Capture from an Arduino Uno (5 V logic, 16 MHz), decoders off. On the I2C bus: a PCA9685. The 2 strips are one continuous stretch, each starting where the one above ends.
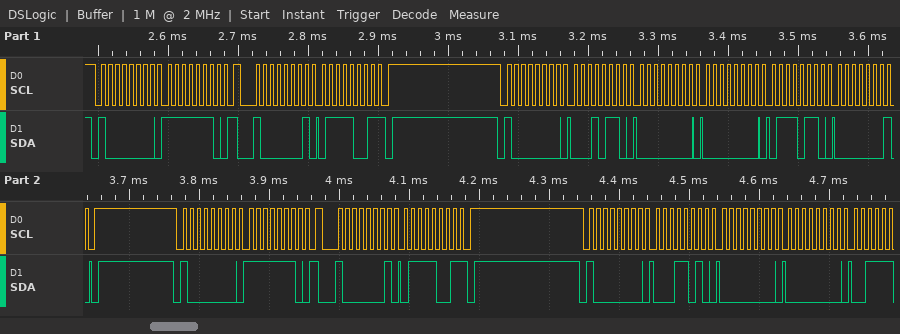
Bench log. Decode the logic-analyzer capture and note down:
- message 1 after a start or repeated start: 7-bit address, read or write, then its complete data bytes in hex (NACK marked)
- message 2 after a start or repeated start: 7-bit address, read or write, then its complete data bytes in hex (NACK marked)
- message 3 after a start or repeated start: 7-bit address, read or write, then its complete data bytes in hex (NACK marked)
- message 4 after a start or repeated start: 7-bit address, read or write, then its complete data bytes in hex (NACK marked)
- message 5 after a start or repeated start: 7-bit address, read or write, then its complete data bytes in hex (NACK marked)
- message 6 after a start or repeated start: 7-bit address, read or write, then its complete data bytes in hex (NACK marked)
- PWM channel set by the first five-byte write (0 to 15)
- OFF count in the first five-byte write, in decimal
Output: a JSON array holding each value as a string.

["0x40 write: FE", "0x40 read: 79 NACK", "0x40 write: 16 00 00 76 01", "0x40 write: FE", "0x40 read: 79 NACK", "0x40 write: 1A 00 00", "4", "374"]
